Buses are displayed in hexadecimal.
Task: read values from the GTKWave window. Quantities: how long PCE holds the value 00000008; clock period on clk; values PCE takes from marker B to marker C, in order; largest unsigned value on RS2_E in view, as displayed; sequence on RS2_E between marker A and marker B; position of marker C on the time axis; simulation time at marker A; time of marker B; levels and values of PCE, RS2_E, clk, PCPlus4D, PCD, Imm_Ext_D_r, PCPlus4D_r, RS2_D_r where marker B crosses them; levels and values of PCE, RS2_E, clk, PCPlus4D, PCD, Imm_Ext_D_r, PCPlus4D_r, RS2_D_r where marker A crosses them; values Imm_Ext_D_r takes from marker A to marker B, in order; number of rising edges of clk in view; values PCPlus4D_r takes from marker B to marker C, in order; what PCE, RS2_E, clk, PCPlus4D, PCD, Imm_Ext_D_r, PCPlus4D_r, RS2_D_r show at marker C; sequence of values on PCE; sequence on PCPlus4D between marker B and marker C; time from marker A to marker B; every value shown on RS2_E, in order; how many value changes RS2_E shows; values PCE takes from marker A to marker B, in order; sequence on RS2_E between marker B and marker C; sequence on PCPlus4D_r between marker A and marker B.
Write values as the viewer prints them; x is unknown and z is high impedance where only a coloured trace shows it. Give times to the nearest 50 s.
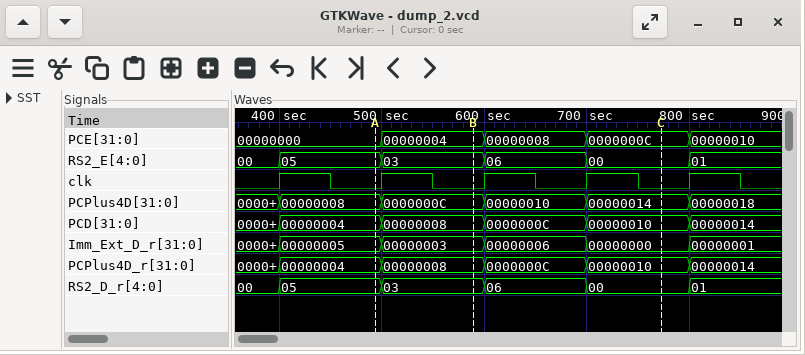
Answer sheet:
100 s
100 s
00000004, 00000008, 0000000C
06
05, 03
750 s
500 s
600 s
PCE=00000004, RS2_E=03, clk=0, PCPlus4D=0000000C, PCD=00000008, Imm_Ext_D_r=00000003, PCPlus4D_r=00000008, RS2_D_r=03
PCE=00000000, RS2_E=05, clk=0, PCPlus4D=00000008, PCD=00000004, Imm_Ext_D_r=00000005, PCPlus4D_r=00000004, RS2_D_r=05
00000005, 00000003
5
00000008, 0000000C, 00000010
PCE=0000000C, RS2_E=00, clk=0, PCPlus4D=00000014, PCD=00000010, Imm_Ext_D_r=00000000, PCPlus4D_r=00000010, RS2_D_r=00
00000000, 00000004, 00000008, 0000000C, 00000010
0000000C, 00000010, 00000014
100 s
00, 05, 03, 06, 00, 01
5
00000000, 00000004
03, 06, 00
00000004, 00000008
